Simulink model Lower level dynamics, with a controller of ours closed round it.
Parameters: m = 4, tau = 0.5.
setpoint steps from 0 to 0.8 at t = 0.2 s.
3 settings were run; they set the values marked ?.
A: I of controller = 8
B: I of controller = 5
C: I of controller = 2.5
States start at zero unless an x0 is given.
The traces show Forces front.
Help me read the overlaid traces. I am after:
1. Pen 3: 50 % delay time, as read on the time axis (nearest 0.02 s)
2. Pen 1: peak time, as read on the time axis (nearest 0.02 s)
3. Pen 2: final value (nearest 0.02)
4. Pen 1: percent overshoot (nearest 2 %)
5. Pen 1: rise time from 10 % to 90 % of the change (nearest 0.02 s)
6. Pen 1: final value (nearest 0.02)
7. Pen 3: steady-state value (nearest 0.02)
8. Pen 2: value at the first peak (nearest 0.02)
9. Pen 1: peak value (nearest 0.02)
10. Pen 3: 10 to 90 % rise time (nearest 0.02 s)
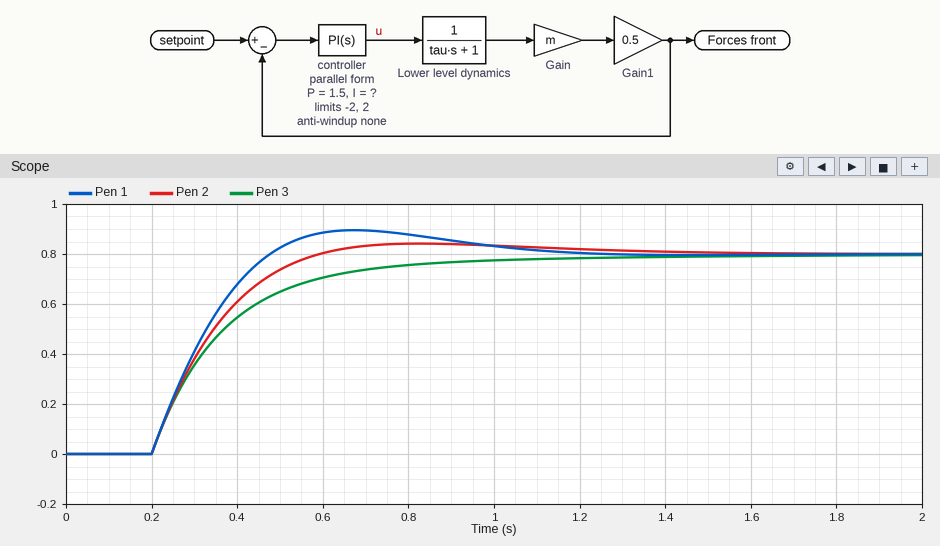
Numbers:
0.32 s
0.68 s
0.80
12 %
0.20 s
0.80
0.80
0.84
0.90
0.42 s
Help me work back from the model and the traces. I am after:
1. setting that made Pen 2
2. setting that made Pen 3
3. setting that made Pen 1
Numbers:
B
C
A
